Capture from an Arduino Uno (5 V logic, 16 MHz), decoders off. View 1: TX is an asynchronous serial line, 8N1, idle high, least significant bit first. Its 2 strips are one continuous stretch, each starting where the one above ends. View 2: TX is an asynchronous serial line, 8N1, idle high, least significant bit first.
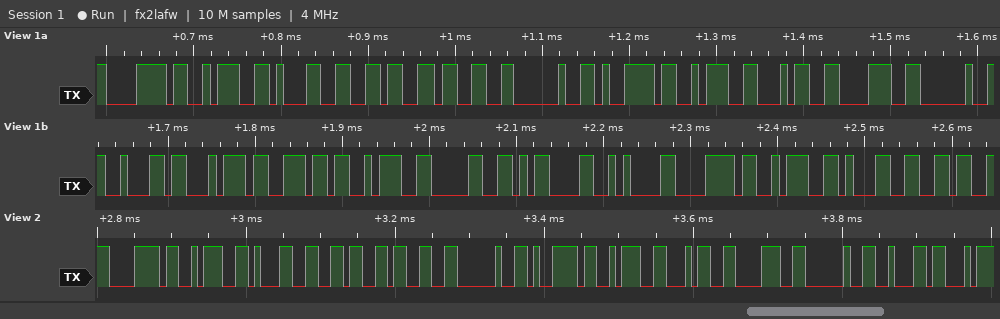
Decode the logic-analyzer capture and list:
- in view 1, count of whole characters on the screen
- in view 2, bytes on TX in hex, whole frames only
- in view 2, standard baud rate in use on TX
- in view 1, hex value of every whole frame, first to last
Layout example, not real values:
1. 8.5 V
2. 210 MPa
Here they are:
1. 22
2. 78 3A 31 36 33 20 79 3A 34 38 20 62
3. 115200 baud
4. 78 3A 31 36 33 20 79 3A 34 38 20 62 74 6E 3A 30 0D 0A 78 3A 31 36
